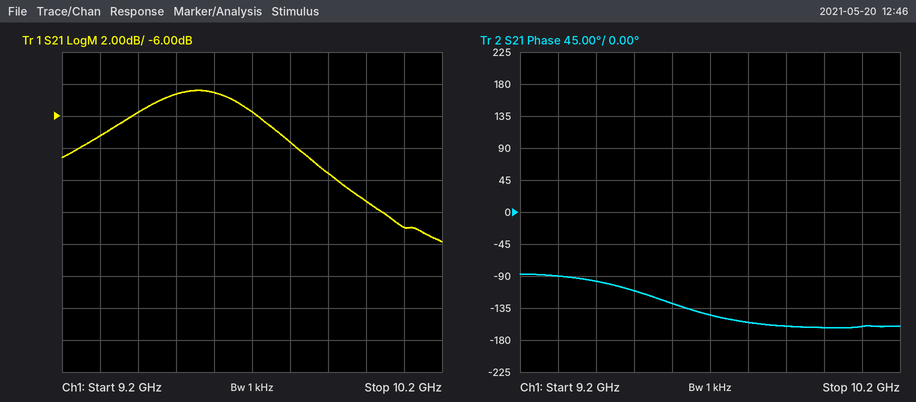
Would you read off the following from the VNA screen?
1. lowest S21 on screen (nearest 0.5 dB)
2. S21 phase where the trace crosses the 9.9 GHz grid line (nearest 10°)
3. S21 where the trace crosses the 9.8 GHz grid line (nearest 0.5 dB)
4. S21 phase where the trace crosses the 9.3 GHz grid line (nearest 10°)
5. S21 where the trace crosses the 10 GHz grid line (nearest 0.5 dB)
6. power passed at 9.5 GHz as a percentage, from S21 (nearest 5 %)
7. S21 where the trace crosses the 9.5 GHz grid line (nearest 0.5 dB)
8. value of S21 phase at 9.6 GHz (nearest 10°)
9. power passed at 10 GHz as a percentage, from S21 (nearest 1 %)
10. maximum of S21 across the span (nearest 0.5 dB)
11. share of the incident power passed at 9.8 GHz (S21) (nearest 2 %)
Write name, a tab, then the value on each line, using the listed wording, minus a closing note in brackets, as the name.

lowest S21 on screen	-14.0 dB
S21 phase where the trace crosses the 9.9 GHz grid line	-160°
S21 where the trace crosses the 9.8 GHz grid line	-7.5 dB
S21 phase where the trace crosses the 9.3 GHz grid line	-90°
S21 where the trace crosses the 10 GHz grid line	-11.5 dB
power passed at 9.5 GHz as a percentage, from S21	35 %
S21 where the trace crosses the 9.5 GHz grid line	-4.5 dB
value of S21 phase at 9.6 GHz	-130°
power passed at 10 GHz as a percentage, from S21	7 %
maximum of S21 across the span	-4.5 dB
share of the incident power passed at 9.8 GHz (S21)	18 %
